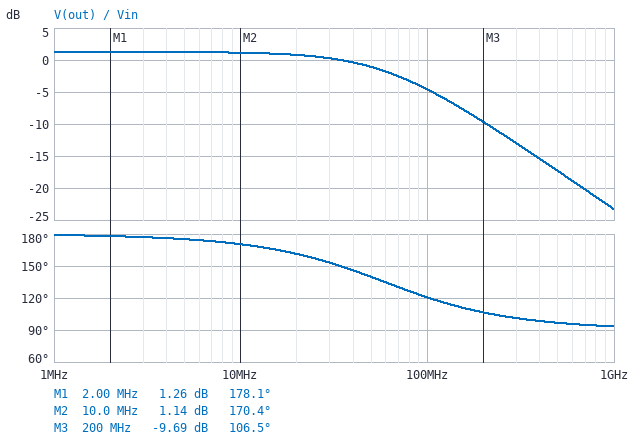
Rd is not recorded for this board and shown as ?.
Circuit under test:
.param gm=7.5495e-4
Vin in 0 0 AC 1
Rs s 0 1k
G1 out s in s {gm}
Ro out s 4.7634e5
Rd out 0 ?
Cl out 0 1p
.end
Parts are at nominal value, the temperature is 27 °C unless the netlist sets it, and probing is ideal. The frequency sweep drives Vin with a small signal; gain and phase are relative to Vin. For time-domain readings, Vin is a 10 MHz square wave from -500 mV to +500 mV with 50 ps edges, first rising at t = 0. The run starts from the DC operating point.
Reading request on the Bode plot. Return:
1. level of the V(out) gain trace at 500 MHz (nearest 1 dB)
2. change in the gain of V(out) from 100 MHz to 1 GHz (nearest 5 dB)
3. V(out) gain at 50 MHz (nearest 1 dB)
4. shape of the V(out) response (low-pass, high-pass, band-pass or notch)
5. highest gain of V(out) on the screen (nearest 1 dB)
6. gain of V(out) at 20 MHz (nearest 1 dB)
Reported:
-17 dB
-20 dB
-1 dB
low-pass
1 dB
1 dB
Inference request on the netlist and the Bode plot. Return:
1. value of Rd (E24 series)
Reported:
2.7 kΩ
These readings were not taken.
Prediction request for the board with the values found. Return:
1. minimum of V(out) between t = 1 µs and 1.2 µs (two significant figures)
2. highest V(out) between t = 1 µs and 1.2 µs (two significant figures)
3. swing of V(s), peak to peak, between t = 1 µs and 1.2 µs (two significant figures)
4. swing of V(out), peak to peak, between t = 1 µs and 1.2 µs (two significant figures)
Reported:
-580 mV
580 mV
430 mV
1.2 V
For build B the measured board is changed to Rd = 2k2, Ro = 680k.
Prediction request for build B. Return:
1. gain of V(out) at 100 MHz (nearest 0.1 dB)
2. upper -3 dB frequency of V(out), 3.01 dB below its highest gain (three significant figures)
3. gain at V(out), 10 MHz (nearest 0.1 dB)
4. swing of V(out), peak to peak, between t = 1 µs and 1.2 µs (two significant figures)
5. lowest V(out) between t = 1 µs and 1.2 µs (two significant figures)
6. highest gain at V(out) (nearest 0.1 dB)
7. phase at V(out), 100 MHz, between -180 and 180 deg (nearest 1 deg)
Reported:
-5.1 dB
72.5 MHz
-0.6 dB
940 mV
-470 mV
-0.5 dB
126 deg
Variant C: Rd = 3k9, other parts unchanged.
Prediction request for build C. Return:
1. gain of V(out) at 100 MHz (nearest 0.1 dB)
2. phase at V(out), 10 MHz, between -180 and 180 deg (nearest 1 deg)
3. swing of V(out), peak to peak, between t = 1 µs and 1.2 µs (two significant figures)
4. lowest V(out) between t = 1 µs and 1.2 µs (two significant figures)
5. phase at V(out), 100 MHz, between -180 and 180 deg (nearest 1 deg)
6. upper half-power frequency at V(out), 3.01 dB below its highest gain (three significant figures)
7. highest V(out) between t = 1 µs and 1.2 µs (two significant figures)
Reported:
-4.0 dB
166 deg
1.7 V
-830 mV
112 deg
41.0 MHz
830 mV
